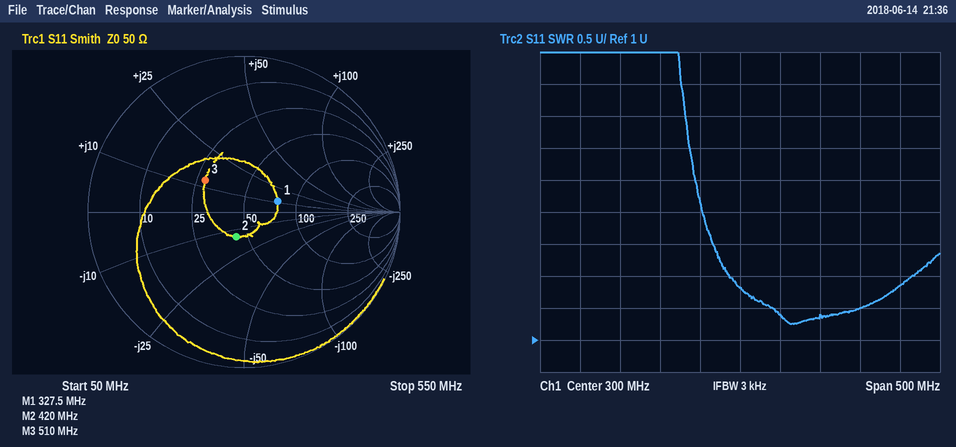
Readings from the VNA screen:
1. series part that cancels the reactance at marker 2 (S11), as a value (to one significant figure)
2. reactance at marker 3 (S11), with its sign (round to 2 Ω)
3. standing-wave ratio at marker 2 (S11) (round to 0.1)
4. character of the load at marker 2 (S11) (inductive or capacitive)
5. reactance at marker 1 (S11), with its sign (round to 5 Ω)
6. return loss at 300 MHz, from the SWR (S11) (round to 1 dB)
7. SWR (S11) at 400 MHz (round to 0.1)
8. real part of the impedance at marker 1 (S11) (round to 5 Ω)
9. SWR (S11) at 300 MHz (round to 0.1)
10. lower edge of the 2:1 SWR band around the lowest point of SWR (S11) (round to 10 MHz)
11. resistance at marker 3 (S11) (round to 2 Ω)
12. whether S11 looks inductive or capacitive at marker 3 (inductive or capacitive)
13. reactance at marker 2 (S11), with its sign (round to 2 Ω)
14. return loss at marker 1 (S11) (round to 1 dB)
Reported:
5 nH
+12 Ω
1.4
capacitive
+10 Ω
11 dB
1.4
75 Ω
1.8
290 MHz
28 Ω
inductive
-14 Ω
13 dB
